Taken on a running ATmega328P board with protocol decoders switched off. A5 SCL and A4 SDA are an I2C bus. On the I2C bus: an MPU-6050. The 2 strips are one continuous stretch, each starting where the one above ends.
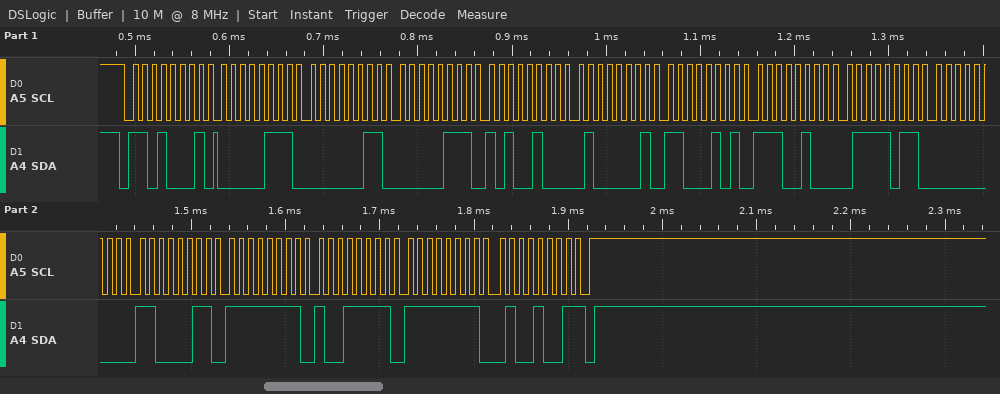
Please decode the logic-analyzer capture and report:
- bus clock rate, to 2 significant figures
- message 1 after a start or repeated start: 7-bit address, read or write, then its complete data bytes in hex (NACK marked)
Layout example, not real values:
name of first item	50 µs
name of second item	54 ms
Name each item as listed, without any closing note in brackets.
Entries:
bus clock rate, to 2 significant figures	100 kHz
message 1 after a start or repeated start: 7-bit address, read or write, then its complete data bytes in hex	0x68 read: 07 03 07 A4 41 C5 E4 7B 00 C3 FF 9F FF 49 NACK
